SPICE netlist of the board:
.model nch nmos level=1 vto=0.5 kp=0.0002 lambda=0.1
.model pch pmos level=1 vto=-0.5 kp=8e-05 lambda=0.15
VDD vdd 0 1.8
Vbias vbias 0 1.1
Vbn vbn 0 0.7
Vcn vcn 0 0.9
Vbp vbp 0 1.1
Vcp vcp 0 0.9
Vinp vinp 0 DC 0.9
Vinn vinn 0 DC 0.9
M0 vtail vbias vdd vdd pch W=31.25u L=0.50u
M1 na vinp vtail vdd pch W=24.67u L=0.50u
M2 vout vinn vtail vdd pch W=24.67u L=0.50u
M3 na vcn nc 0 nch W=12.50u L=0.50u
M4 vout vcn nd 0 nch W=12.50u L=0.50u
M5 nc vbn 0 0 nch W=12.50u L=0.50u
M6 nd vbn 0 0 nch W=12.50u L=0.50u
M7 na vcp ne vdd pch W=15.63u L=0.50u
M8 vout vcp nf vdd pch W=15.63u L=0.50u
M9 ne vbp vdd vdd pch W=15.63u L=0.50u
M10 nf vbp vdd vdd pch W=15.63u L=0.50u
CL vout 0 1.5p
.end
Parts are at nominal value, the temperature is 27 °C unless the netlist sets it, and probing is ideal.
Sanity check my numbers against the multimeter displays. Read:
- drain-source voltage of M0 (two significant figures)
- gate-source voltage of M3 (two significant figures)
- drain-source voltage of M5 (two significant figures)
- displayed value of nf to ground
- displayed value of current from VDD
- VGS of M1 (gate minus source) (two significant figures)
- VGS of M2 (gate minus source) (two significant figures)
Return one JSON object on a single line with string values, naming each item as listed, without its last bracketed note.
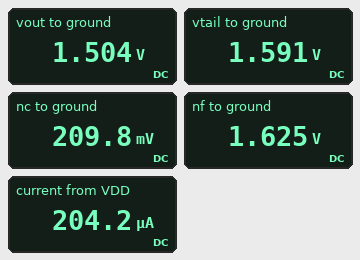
{"drain-source voltage of M0": "-210 mV", "gate-source voltage of M3": "690 mV", "drain-source voltage of M5": "210 mV", "displayed value of nf to ground": "1.625 V", "displayed value of current from VDD": "204.2 µA", "VGS of M1 (gate minus source)": "-690 mV", "VGS of M2 (gate minus source)": "-690 mV"}
